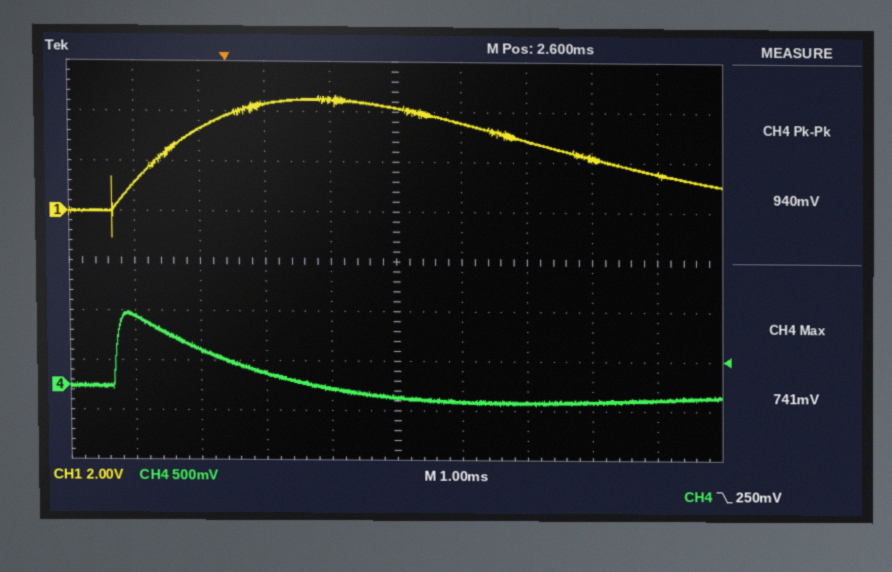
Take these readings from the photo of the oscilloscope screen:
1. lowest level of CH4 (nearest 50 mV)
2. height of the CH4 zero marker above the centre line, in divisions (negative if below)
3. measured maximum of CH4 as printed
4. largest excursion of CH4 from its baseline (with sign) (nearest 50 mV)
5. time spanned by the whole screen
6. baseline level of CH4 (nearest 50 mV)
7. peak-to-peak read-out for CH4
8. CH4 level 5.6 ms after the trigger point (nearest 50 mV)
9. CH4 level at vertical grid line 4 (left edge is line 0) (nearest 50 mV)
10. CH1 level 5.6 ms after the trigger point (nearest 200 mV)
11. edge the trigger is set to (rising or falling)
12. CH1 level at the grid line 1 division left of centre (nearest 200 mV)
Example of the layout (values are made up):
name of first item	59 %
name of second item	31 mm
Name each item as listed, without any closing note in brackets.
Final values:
lowest level of CH4	-200 mV
height of the CH4 zero marker above the centre line, in divisions	-2.5 div
measured maximum of CH4 as printed	741 mV
largest excursion of CH4 from its baseline (with sign)	+900 mV
time spanned by the whole screen	10 ms
baseline level of CH4	-150 mV
peak-to-peak read-out for CH4	940 mV
CH4 level 5.6 ms after the trigger point	-150 mV
CH4 level at vertical grid line 4 (left edge is line 0)	-50 mV
CH1 level 5.6 ms after the trigger point	2.2 V
edge the trigger is set to	falling
CH1 level at the grid line 1 division left of centre	4.4 V
